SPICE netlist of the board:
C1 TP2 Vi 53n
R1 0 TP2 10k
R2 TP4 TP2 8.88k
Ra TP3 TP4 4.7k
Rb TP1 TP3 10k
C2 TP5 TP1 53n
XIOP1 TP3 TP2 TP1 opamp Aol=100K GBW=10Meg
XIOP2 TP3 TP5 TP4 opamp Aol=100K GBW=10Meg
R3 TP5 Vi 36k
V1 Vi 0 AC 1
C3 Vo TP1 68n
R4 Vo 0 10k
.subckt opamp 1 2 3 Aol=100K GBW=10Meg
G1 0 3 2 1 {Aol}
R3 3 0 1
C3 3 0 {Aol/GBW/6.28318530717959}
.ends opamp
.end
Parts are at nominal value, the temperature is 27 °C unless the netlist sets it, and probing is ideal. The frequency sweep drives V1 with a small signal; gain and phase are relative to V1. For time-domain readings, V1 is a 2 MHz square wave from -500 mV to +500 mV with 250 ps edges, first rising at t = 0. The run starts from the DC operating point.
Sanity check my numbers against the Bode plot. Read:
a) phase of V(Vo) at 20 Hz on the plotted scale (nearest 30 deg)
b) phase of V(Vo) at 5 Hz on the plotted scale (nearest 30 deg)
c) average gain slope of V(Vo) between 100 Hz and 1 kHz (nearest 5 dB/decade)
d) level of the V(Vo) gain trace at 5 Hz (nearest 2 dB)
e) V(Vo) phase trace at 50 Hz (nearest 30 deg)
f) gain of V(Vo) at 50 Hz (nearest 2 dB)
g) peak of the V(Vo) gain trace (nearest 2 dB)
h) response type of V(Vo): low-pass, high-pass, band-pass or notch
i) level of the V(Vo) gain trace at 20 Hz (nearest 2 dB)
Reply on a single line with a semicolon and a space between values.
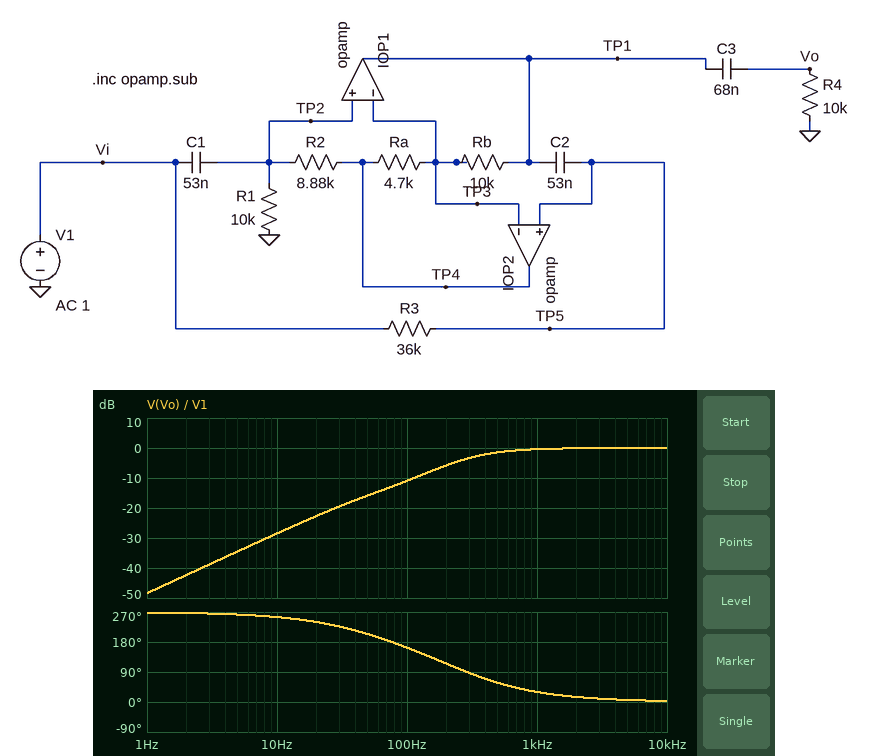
240 deg; 270 deg; 10 dB/decade; -34 dB; 210 deg; -16 dB; 0 dB; high-pass; -22 dB
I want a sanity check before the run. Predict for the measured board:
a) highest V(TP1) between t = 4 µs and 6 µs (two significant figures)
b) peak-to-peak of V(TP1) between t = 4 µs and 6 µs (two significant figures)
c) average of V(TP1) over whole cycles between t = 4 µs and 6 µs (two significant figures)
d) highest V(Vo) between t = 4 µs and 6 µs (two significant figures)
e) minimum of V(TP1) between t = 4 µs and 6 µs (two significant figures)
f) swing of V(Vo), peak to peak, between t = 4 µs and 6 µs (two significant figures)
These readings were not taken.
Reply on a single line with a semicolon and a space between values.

1.7 V; 1.5 V; 940 mV; 1.2 V; 190 mV; 1.5 V
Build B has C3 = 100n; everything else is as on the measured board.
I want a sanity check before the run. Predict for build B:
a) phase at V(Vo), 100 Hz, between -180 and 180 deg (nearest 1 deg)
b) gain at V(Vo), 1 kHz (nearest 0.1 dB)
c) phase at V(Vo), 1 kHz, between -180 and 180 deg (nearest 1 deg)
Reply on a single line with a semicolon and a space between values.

154 deg; -0.3 dB; 26 deg
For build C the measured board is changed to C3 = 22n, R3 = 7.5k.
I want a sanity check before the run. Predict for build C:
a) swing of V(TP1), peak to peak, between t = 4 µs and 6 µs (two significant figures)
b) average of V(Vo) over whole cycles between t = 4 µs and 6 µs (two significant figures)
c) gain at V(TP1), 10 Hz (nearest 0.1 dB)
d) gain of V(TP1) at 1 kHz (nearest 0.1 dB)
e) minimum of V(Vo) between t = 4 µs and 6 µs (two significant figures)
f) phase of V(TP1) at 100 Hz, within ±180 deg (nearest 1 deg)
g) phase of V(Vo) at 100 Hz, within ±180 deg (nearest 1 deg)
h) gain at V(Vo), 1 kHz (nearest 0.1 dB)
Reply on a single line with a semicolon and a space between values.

1.5 V; 480 mV; -1.0 dB; 0.6 dB; -270 mV; 151 deg; -127 deg; -1.2 dB
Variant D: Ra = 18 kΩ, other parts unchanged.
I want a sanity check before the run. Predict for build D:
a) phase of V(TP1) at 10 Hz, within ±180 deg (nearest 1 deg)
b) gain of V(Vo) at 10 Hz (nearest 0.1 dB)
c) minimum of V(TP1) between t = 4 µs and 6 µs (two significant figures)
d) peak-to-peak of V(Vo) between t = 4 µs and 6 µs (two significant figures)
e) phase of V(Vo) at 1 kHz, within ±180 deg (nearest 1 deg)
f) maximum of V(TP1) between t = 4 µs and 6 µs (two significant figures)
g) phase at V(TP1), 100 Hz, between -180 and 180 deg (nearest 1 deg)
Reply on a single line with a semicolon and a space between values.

-3 deg; -33.3 dB; -430 mV; 1.3 V; 31 deg; 910 mV; -36 deg
